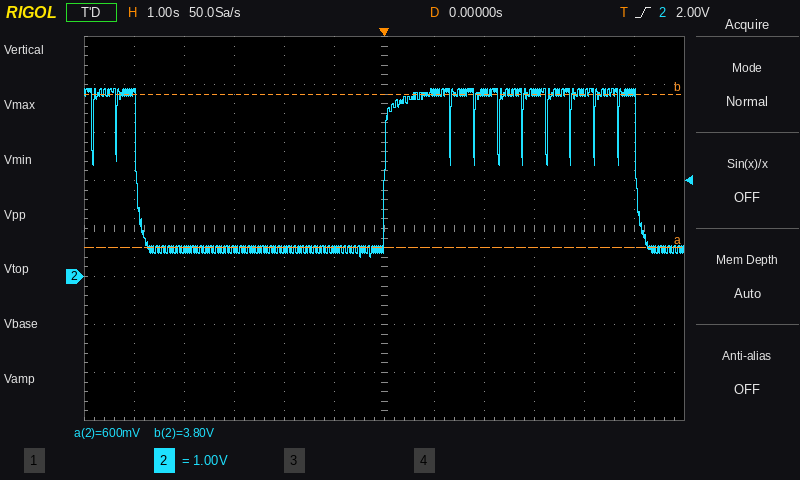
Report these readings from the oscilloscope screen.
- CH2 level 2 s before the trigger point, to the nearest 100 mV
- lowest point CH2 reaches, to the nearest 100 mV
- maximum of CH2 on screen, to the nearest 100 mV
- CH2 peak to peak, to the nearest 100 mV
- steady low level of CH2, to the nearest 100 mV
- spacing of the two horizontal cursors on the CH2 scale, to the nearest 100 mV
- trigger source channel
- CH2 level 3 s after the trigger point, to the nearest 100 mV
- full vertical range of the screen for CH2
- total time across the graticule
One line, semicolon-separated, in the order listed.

600 mV; 400 mV; 3.9 V; 3.5 V; 600 mV; 3.2 V; CH2; 3.8 V; 8 V; 12 s
